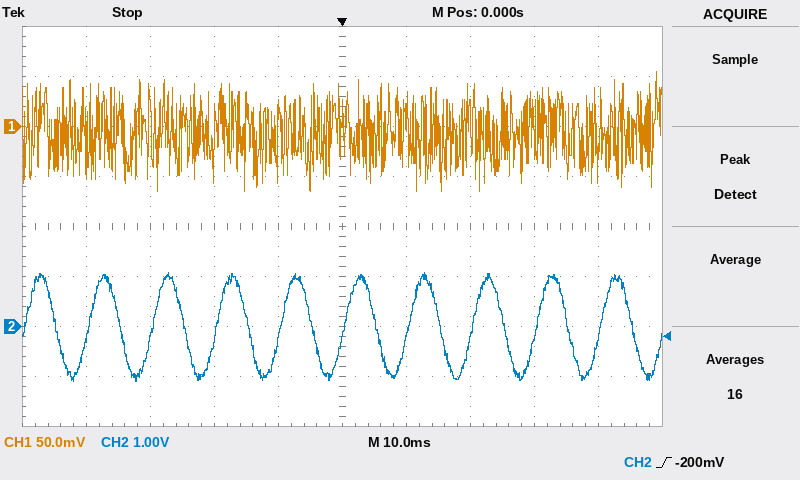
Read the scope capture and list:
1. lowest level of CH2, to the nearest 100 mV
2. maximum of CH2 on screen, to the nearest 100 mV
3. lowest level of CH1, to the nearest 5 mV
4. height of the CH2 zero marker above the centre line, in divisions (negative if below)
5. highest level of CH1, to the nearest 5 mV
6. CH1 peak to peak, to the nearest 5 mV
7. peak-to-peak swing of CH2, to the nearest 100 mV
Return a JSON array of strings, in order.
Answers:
["-1.1 V", "1.1 V", "-65 mV", "-2.0 div", "55 mV", "120 mV", "2.2 V"]
